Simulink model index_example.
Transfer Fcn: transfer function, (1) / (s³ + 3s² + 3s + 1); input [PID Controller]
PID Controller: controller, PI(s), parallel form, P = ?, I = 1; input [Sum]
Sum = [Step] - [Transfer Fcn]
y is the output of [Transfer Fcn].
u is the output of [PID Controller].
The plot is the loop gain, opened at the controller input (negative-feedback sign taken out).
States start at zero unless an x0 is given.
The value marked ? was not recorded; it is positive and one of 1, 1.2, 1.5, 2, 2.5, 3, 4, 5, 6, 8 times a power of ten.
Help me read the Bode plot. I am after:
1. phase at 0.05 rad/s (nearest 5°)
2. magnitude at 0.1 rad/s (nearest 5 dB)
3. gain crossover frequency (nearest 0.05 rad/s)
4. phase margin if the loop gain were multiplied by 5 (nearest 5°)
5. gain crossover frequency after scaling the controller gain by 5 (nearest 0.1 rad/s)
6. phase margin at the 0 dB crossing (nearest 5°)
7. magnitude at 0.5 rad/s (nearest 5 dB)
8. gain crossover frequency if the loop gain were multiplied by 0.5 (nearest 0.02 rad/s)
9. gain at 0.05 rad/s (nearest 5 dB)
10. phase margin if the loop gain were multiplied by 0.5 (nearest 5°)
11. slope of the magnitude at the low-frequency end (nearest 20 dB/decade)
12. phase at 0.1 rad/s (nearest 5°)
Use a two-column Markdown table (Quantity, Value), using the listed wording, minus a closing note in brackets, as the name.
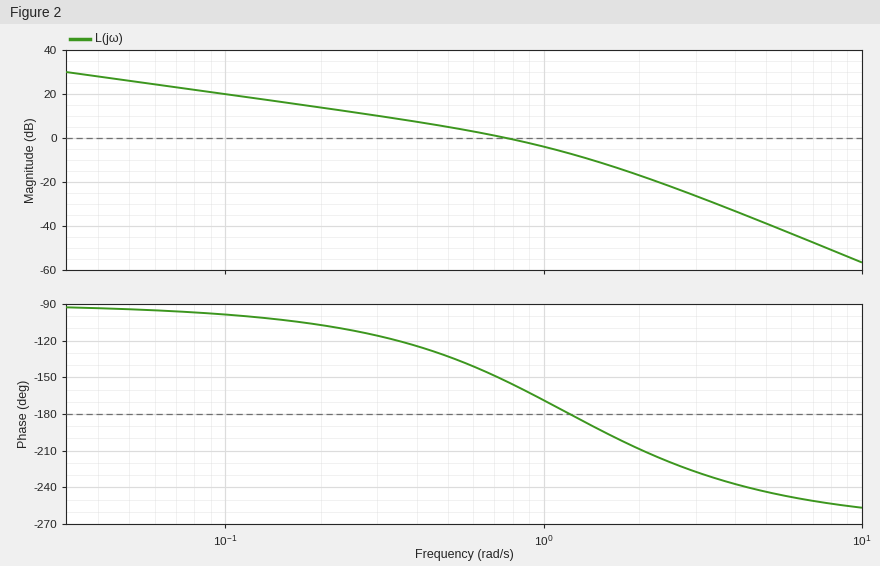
| Quantity | Value |
|---|---|
| phase at 0.05 rad/s | -95° |
| magnitude at 0.1 rad/s | 20 dB |
| gain crossover frequency | 0.75 rad/s |
| phase margin if the loop gain were multiplied by 5 | -20° |
| gain crossover frequency after scaling the controller gain by 5 | 1.7 rad/s |
| phase margin at the 0 dB crossing | 25° |
| magnitude at 0.5 rad/s | 5 dB |
| gain crossover frequency if the loop gain were multiplied by 0.5 | 0.46 rad/s |
| gain at 0.05 rad/s | 25 dB |
| phase margin if the loop gain were multiplied by 0.5 | 50° |
| slope of the magnitude at the low-frequency end | -20 dB/decade |
| phase at 0.1 rad/s | -100° |
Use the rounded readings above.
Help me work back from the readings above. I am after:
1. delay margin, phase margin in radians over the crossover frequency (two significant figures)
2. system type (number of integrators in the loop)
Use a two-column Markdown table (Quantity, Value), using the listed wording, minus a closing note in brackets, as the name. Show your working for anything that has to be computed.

| Quantity | Value |
|---|---|
| delay margin, phase margin in radians over the crossover frequency | 25 × π / 180 / 0.75 = 0.58 s |
| system type | 1 |
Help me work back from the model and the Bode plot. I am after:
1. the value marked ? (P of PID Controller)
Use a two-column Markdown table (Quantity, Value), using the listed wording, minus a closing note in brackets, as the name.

| Quantity | Value |
|---|---|
| the value marked ? | 1.5 |
